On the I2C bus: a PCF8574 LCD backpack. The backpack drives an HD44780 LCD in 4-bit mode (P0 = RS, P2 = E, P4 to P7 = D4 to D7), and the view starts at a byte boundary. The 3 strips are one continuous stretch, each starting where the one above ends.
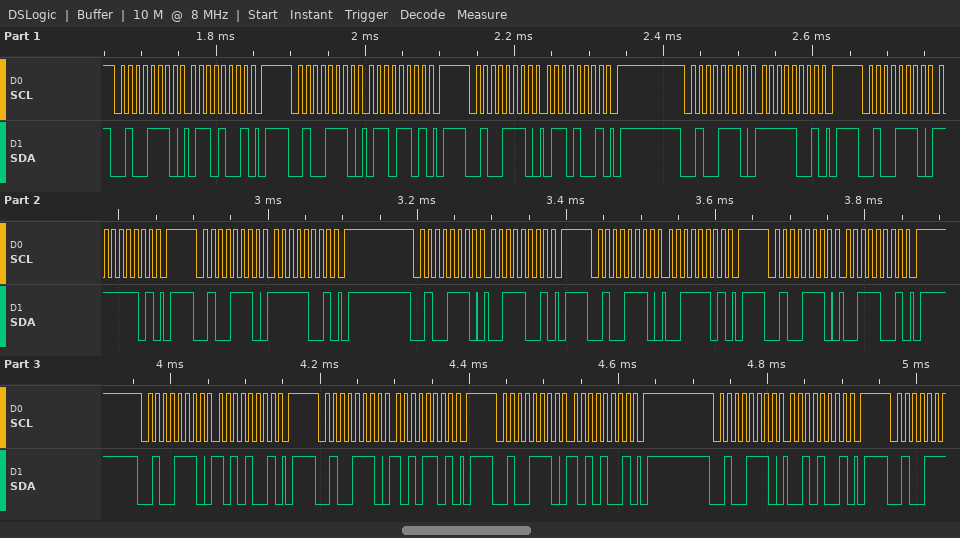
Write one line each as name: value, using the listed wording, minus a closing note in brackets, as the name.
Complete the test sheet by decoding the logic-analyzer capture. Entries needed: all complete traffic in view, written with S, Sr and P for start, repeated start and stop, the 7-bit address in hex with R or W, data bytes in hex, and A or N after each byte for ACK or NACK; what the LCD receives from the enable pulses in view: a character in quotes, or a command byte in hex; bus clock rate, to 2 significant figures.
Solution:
all complete traffic in view, written with S, Sr and P for start, repeated start and stop, the 7-bit address in hex with R or W, data bytes in hex, and A or N after each byte for ACK or NACK: S 27W A 69 A P S 27W A 6D A P S 27W A 69 A P S 27W A F9 A P S 27W A FD A P S 27W A F9 A P S 27W A 39 A P S 27W A 3D A P S 27W A 39 A P S 27W A A9 A P S 27W A AD A P S 27W A A9 A P S 27W A 29 A P
what the LCD receives from the enable pulses in view: a character in quotes, or a command byte in hex: 'o' ':'
bus clock rate, to 2 significant figures: 100 kHz
